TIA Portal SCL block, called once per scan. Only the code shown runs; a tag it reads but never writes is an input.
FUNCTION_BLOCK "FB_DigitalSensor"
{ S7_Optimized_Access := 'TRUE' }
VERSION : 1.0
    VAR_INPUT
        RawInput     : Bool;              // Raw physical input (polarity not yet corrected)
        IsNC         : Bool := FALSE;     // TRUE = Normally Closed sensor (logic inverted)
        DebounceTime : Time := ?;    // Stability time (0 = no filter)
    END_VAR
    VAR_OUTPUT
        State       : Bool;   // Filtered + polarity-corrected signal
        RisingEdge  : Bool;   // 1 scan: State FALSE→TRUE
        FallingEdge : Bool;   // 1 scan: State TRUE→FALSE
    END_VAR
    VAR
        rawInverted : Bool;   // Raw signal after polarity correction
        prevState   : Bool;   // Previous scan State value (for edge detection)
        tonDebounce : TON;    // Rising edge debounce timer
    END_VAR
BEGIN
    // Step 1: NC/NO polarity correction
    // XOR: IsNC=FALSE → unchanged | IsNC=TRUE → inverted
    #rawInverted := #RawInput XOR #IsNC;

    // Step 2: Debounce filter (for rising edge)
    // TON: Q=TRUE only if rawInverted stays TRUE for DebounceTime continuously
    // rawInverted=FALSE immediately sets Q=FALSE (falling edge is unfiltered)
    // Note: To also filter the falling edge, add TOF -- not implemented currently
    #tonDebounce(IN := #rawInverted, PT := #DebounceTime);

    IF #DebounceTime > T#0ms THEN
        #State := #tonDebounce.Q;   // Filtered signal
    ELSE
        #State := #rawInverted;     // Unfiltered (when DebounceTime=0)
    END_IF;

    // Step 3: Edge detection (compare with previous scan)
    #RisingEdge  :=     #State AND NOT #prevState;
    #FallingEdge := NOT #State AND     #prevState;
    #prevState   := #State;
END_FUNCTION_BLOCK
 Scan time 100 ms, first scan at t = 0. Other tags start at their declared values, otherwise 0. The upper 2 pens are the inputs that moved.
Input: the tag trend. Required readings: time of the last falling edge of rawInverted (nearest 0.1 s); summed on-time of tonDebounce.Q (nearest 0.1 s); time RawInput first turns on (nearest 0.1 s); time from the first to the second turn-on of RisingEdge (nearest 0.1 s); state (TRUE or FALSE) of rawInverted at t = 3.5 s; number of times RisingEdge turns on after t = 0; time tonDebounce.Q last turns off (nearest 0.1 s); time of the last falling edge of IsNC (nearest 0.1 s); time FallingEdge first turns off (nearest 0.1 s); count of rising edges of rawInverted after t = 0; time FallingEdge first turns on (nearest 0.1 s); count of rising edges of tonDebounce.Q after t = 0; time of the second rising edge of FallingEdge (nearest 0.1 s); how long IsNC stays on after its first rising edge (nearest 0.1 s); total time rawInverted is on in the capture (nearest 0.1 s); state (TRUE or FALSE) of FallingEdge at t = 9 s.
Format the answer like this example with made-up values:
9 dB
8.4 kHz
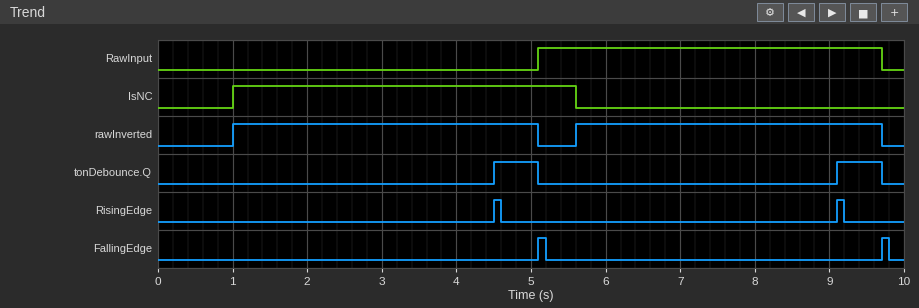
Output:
9.7 s
1.2 s
5.1 s
4.6 s
TRUE
2
9.7 s
5.6 s
5.2 s
2
5.1 s
2
9.7 s
4.6 s
8.2 s
FALSE
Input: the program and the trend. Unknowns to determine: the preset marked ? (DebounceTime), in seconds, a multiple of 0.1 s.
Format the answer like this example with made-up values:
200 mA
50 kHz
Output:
3.5 s
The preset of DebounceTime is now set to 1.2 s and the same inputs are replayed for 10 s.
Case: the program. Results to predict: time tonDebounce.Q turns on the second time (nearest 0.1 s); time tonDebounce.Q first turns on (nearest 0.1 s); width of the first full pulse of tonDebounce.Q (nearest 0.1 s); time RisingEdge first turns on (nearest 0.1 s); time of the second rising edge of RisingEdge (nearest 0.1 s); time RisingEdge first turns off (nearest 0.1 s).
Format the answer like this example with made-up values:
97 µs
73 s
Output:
6.8 s
2.2 s
2.9 s
2.2 s
6.8 s
2.3 s
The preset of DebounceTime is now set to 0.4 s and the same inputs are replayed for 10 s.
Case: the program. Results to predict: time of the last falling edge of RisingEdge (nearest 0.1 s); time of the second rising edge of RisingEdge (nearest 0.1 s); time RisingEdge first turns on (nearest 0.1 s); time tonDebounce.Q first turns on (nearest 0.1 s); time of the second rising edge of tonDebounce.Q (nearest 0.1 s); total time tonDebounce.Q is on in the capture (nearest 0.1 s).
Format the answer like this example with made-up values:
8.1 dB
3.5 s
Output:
6.1 s
6.0 s
1.4 s
1.4 s
6.0 s
7.4 s
